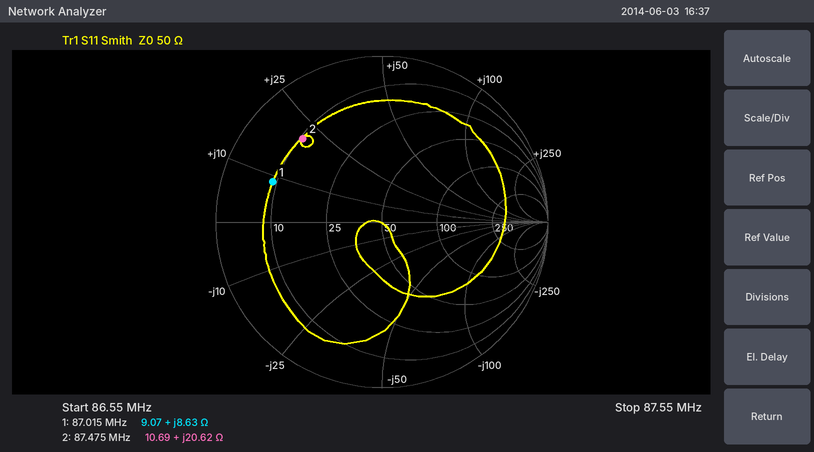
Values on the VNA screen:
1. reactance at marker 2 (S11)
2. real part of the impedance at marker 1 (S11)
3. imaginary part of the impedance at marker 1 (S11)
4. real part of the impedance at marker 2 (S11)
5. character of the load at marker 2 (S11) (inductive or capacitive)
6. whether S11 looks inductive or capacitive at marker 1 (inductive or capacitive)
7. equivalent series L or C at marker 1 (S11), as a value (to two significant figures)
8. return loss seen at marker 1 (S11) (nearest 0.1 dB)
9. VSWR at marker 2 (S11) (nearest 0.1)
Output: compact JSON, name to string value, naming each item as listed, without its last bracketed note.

{"reactance at marker 2": "+20.62 Ω", "real part of the impedance at marker 1": "9.07 Ω", "imaginary part of the impedance at marker 1": "+8.63 Ω", "real part of the impedance at marker 2": "10.69 Ω", "character of the load at marker 2 (S11)": "inductive", "whether S11 looks inductive or capacitive at marker 1": "inductive", "equivalent series L or C at marker 1 (S11), as a value": "16 nH", "return loss seen at marker 1 (S11)": "3.1 dB", "VSWR at marker 2 (S11)": "5.5"}
